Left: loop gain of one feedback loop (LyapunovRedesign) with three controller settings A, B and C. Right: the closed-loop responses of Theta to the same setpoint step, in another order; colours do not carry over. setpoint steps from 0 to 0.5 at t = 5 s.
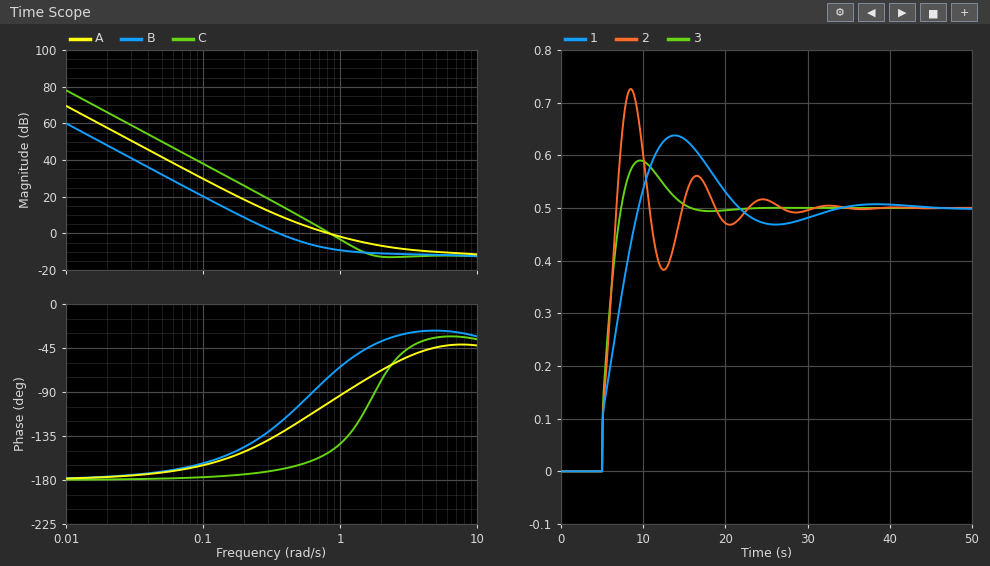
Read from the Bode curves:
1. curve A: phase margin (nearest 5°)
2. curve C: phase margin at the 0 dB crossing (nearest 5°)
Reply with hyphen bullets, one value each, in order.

- 80°
- 30°
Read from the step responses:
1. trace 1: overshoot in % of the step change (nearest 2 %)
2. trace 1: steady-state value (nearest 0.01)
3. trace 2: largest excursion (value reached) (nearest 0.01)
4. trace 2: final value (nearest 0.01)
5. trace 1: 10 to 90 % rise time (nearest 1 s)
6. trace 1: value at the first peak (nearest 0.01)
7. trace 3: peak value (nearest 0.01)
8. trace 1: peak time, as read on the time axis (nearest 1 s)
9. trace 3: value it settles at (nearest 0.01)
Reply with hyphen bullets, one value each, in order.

- 28 %
- 0.50
- 0.73
- 0.50
- 4 s
- 0.64
- 0.59
- 14 s
- 0.50
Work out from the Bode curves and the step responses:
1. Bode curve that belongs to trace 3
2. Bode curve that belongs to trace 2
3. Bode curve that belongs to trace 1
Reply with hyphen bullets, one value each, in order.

- A
- C
- B
